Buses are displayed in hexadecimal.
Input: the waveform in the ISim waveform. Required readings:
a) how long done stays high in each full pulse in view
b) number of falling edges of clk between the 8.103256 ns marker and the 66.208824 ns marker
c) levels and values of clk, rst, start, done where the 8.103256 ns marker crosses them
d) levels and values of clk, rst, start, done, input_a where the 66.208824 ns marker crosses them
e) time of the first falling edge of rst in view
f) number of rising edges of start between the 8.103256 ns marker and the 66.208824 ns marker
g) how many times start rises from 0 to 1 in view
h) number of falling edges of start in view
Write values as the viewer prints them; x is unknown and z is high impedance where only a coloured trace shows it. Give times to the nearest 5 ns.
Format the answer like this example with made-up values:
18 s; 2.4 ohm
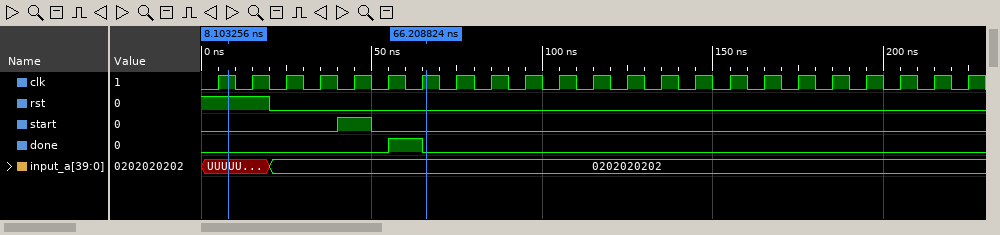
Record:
10 ns; 6; clk=1, rst=1, start=0, done=0; clk=1, rst=0, start=0, done=0, input_a=0202020202; 20 ns; 1; 1; 1
